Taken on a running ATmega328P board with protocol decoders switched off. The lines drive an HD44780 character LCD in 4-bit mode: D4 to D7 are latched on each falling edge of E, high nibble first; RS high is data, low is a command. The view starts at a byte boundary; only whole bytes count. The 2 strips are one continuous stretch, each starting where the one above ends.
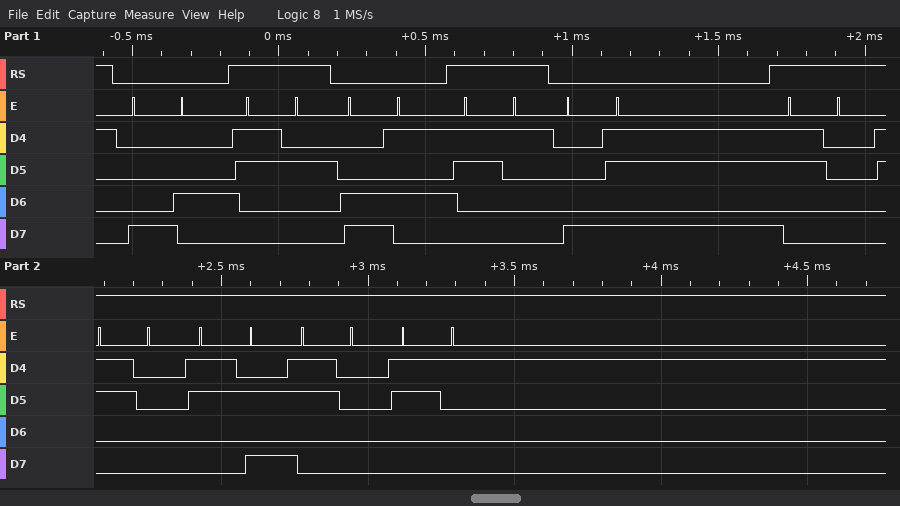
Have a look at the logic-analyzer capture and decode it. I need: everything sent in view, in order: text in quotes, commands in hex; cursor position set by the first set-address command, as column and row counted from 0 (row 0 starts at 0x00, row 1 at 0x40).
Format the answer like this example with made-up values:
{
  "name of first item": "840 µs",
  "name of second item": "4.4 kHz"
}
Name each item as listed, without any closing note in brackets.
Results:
{
  "everything sent in view, in order: text in quotes, commands in hex": "0x84 \"2\" 0xC5 \"1\" 0x8B \"00:01\"",
  "cursor position set by the first set-address command, as column and row counted from 0": "column 4, row 0"
}
